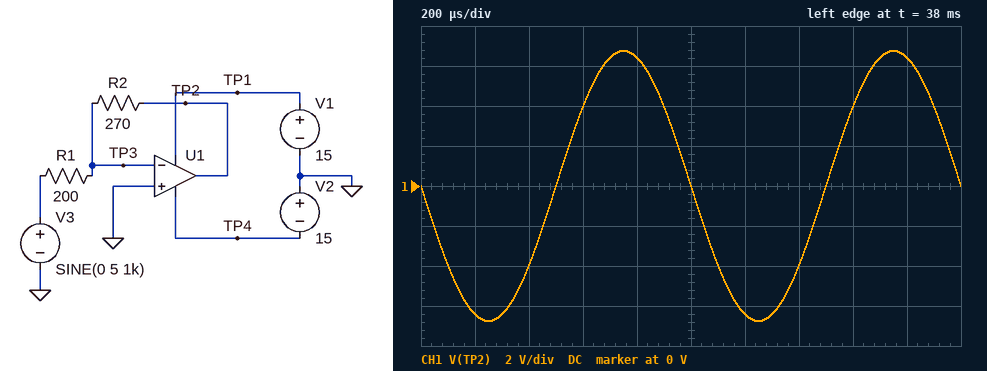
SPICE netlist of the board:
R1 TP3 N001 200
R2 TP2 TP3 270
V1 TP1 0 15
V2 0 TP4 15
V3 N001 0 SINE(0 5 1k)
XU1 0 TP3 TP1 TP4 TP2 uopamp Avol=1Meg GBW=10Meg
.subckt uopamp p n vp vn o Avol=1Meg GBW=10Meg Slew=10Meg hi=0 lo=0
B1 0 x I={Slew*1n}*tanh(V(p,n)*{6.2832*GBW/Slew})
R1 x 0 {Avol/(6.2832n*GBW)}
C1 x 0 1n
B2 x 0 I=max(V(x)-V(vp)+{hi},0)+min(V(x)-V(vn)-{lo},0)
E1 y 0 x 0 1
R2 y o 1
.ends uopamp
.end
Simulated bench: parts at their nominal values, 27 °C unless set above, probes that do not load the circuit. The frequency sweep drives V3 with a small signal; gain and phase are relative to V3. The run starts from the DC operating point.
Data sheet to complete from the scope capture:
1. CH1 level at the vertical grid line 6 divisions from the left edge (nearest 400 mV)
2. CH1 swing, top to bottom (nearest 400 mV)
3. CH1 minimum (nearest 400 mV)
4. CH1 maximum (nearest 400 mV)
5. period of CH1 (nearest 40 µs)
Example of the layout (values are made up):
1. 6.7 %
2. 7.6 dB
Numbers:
1. -6.4 V
2. 13.6 V
3. -6.8 V
4. 6.8 V
5. 1.00 ms
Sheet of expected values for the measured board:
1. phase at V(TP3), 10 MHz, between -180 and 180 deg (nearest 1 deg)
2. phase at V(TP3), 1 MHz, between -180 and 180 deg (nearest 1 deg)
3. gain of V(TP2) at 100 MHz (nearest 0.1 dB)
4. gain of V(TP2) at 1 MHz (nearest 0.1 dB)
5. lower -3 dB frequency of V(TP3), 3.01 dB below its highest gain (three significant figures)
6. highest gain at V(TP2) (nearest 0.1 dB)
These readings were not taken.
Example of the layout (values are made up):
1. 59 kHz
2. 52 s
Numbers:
1. 23 deg
2. 77 deg
3. -24.8 dB
4. 2.4 dB
5. 4.25 MHz
6. 2.6 dB
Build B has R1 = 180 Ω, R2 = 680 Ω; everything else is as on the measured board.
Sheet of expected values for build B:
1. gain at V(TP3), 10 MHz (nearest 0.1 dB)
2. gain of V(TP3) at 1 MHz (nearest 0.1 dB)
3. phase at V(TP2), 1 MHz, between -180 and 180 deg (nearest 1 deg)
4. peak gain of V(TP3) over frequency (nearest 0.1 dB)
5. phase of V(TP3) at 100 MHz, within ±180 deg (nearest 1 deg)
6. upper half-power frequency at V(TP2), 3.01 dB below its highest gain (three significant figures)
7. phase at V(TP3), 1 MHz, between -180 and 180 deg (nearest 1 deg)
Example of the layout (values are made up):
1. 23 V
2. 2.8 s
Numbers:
1. -2.2 dB
2. -9.3 dB
3. 154 deg
4. -2.0 dB
5. 1 deg
6. 2.09 MHz
7. 64 deg
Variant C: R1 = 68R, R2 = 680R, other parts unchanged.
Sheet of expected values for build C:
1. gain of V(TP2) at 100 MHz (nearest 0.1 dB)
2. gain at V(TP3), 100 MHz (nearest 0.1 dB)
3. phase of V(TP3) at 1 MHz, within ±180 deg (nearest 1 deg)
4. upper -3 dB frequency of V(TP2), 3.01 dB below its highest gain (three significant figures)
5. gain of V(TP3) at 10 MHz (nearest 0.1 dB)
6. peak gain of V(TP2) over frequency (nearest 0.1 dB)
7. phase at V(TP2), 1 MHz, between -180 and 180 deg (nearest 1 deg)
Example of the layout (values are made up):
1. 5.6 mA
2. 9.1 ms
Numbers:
1. -20.8 dB
2. -0.8 dB
3. 42 deg
4. 908 kHz
5. -0.9 dB
6. 20.0 dB
7. 132 deg
